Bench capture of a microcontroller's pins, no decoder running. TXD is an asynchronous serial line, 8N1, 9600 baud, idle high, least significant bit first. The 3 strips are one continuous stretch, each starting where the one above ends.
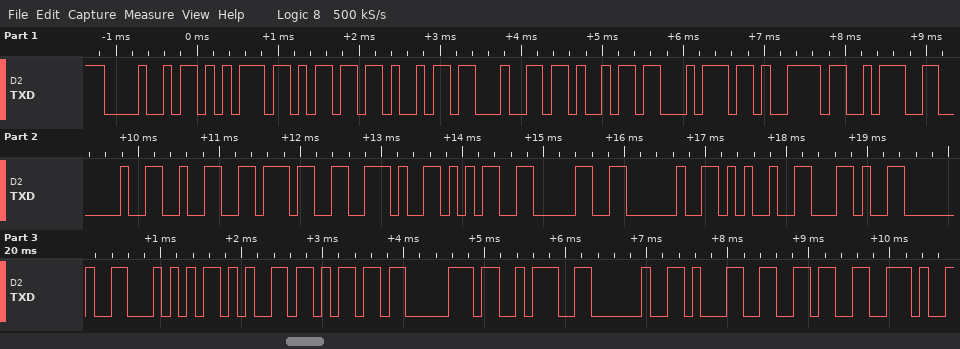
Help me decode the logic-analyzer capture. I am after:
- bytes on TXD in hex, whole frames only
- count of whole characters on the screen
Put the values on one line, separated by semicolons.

0x48 0x75 0x6D 0x69 0x64 0x69 0x74 0x79 0x3A 0x20 0x32 0x37 0x2E 0x35 0x30 0x20 0x25 0x2C 0x20 0x54 0x65 0x6D 0x70 0x3A 0x20 0x31 0x36 0x2E; 28
